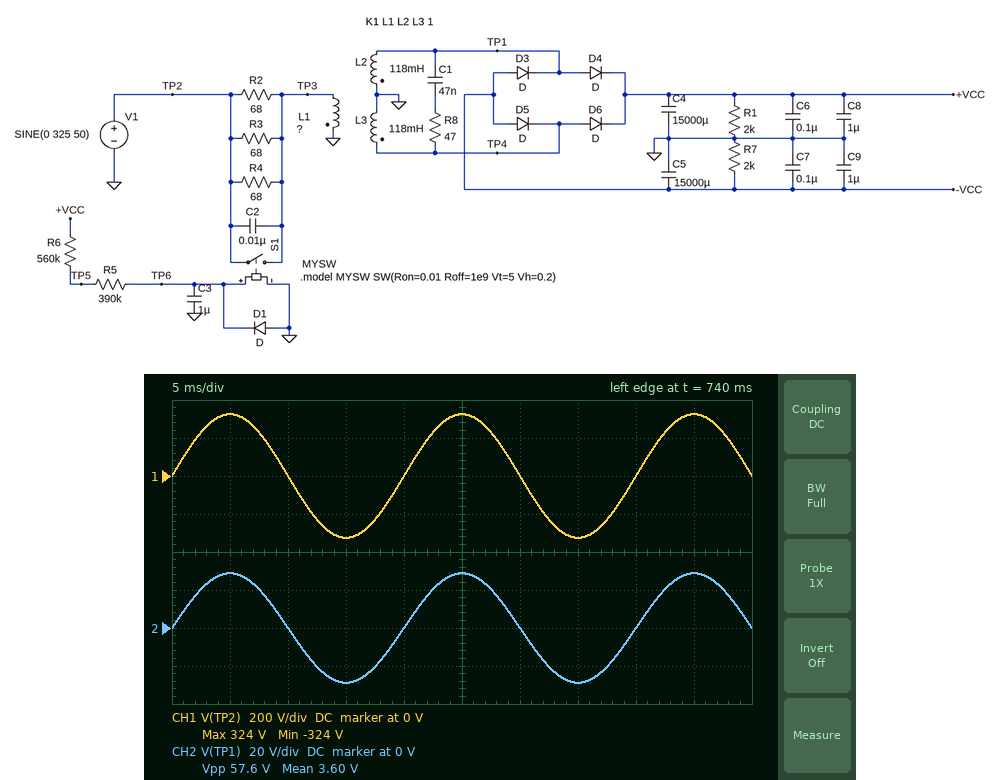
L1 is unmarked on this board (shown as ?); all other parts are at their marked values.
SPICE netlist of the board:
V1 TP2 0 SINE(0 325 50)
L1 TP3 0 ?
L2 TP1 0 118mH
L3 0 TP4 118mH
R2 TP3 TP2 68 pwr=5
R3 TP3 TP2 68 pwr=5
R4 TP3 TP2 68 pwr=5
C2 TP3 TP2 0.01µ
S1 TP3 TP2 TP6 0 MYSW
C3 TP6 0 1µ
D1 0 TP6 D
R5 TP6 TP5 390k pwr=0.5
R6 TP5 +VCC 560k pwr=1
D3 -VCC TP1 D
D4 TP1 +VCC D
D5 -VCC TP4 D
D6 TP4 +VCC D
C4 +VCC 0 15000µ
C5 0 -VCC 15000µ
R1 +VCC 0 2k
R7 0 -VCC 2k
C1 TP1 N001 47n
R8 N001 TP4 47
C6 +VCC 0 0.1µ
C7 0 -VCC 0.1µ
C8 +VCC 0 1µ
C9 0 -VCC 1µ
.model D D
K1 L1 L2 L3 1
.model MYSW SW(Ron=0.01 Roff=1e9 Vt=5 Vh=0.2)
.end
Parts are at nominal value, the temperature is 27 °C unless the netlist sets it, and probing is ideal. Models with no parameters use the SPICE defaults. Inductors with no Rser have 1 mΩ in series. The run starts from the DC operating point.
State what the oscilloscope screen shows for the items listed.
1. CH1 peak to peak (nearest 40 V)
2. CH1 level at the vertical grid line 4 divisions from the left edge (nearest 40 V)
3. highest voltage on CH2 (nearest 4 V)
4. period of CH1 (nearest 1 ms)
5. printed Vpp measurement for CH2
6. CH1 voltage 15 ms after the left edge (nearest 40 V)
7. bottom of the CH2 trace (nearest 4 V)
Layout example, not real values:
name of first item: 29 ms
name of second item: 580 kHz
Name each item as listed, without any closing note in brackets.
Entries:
CH1 peak to peak: 640 V
CH1 level at the vertical grid line 4 divisions from the left edge: 0 V
highest voltage on CH2: 28 V
period of CH1: 20 ms
printed Vpp measurement for CH2: 57.6 V
CH1 voltage 15 ms after the left edge: -320 V
bottom of the CH2 trace: -28 V
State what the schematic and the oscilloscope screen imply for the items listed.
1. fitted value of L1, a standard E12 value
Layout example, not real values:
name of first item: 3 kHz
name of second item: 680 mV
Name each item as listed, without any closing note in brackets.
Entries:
fitted value of L1, a standard E12 value: 15 H
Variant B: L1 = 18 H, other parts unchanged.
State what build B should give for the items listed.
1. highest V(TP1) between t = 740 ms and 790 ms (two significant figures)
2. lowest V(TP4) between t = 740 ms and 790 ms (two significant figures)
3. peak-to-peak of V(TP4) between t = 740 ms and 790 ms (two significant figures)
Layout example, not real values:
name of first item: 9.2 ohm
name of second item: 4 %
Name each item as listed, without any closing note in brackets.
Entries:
highest V(TP1) between t = 740 ms and 790 ms: 26 V
lowest V(TP4) between t = 740 ms and 790 ms: -26 V
peak-to-peak of V(TP4) between t = 740 ms and 790 ms: 53 V
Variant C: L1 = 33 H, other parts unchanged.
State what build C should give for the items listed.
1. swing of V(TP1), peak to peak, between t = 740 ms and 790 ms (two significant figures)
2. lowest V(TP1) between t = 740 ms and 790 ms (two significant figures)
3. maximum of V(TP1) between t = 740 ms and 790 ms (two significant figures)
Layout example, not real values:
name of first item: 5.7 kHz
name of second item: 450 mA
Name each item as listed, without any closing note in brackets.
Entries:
swing of V(TP1), peak to peak, between t = 740 ms and 790 ms: 39 V
lowest V(TP1) between t = 740 ms and 790 ms: -19 V
maximum of V(TP1) between t = 740 ms and 790 ms: 19 V
